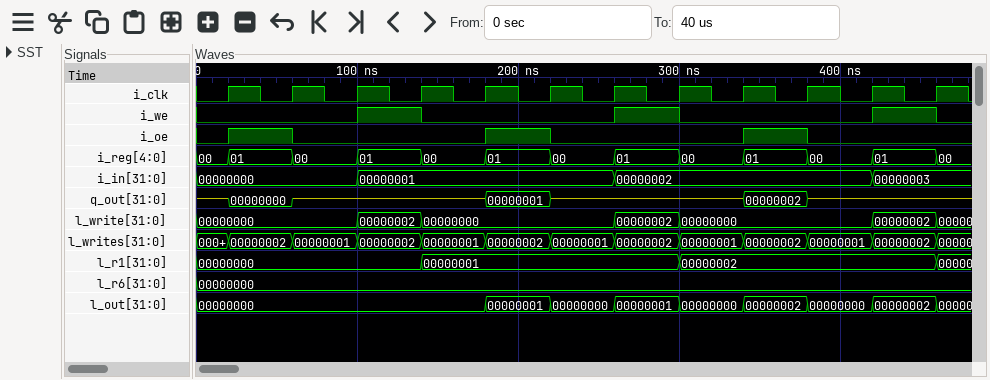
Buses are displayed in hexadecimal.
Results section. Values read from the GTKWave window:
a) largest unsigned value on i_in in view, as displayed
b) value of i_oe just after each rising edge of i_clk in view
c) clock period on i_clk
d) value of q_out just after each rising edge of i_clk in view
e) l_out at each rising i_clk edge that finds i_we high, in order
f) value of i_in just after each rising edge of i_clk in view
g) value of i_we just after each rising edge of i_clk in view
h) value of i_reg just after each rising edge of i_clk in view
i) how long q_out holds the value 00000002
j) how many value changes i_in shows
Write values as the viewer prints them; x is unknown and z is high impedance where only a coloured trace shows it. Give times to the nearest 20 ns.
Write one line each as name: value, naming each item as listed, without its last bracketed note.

largest unsigned value on i_in in view, as displayed: 00000003
value of i_oe just after each rising edge of i_clk in view: 1 0 0 0 1 0 0 0 1 0 0 0
clock period on i_clk: 40 ns
value of q_out just after each rising edge of i_clk in view: 00000000, z, z, z, 00000001, z, z, z, 00000002, z, z, z
l_out at each rising i_clk edge that finds i_we high, in order: 00000000, 00000001, 00000002
value of i_in just after each rising edge of i_clk in view: 00000000, 00000000, 00000001, 00000001, 00000001, 00000001, 00000002, 00000002, 00000002, 00000002, 00000003, 00000003
value of i_we just after each rising edge of i_clk in view: 0 0 1 0 0 0 1 0 0 0 1 0
value of i_reg just after each rising edge of i_clk in view: 01, 00, 01, 00, 01, 00, 01, 00, 01, 00, 01, 00
how long q_out holds the value 00000002: 40 ns
how many value changes i_in shows: 3
